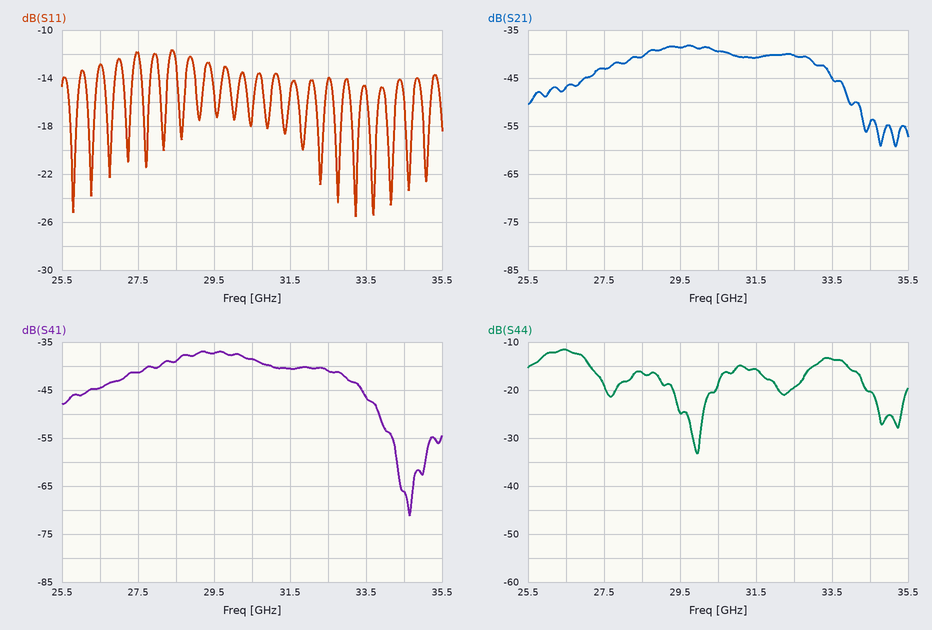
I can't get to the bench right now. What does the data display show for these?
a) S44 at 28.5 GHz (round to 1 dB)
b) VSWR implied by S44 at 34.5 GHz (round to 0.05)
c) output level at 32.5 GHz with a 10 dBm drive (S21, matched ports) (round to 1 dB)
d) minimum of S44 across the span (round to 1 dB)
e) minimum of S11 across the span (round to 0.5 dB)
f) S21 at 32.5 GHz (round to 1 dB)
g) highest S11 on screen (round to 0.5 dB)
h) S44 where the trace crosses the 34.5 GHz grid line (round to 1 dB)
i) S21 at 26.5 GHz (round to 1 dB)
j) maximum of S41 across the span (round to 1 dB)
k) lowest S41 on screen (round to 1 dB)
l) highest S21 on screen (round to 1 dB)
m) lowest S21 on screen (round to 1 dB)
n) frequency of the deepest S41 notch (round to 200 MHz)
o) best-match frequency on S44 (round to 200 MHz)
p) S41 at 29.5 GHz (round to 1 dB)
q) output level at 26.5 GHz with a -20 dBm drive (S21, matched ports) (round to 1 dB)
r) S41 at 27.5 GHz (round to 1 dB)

-16 dB
1.20
-30 dBm
-33 dB
-25.5 dB
-40 dB
-11.5 dB
-20 dB
-47 dB
-37 dB
-71 dB
-38 dB
-59 dB
34.6 GHz
30.0 GHz
-37 dB
-67 dBm
-41 dB
